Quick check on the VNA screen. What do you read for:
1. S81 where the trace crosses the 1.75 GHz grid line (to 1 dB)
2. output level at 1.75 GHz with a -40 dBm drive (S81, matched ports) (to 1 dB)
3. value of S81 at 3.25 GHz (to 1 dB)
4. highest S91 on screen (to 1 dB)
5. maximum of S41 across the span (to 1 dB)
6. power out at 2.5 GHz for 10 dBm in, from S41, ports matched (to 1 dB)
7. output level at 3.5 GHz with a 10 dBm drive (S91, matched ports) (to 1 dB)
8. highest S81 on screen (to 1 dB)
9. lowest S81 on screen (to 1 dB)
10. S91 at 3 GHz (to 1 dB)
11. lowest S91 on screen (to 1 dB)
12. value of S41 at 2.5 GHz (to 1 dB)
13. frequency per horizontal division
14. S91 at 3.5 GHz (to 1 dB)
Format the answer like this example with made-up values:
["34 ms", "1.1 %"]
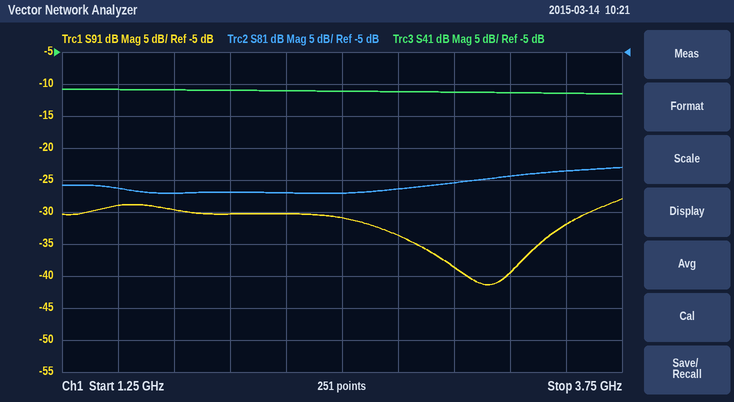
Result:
["-27 dB", "-67 dBm", "-24 dB", "-28 dB", "-11 dB", "-1 dBm", "-22 dBm", "-23 dB", "-27 dB", "-39 dB", "-41 dB", "-11 dB", "250 MHz", "-32 dB"]
